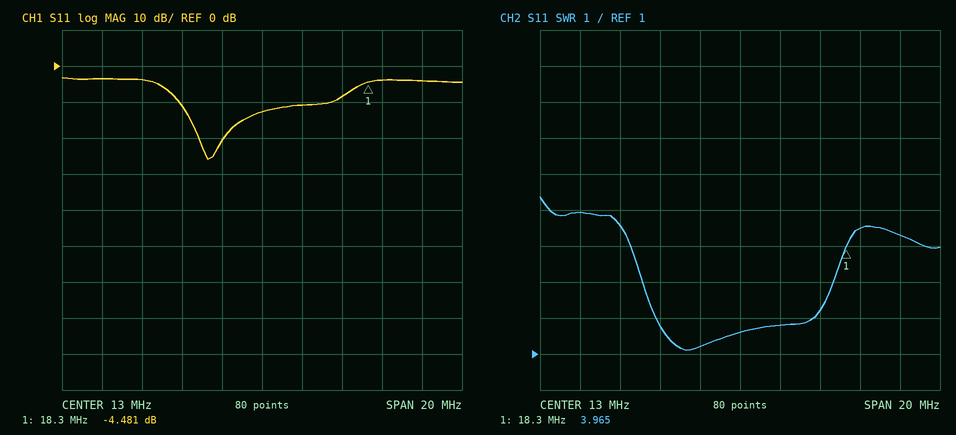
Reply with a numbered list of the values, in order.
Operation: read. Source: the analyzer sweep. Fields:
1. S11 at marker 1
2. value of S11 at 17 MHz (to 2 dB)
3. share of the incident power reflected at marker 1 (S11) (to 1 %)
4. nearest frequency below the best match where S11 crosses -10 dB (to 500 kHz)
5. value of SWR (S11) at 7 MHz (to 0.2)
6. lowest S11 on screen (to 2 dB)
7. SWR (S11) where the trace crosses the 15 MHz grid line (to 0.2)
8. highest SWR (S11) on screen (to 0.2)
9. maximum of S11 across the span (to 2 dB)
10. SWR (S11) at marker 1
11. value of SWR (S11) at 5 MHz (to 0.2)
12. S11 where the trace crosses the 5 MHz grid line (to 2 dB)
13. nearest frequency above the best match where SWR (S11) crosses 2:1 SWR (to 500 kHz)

1. -4.481 dB
2. -8 dB
3. 36 %
4. 9.0 MHz
5. 4.6
6. -26 dB
7. 1.8
8. 5.4
9. -4 dB
10. 3.965
11. 5.0
12. -4 dB
13. 16.5 MHz
